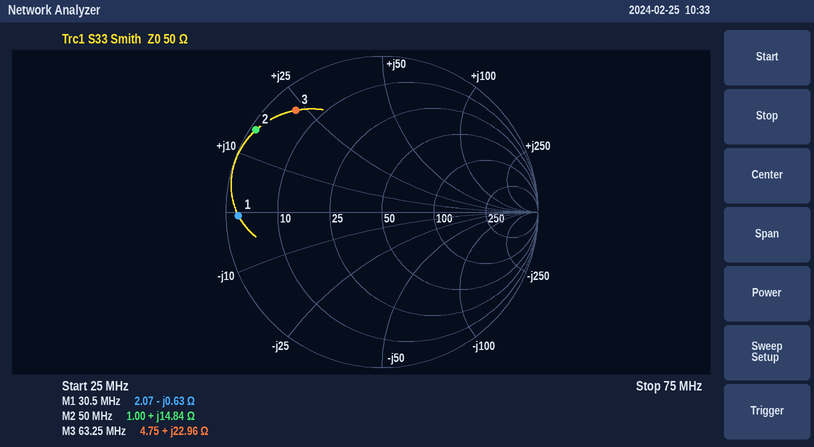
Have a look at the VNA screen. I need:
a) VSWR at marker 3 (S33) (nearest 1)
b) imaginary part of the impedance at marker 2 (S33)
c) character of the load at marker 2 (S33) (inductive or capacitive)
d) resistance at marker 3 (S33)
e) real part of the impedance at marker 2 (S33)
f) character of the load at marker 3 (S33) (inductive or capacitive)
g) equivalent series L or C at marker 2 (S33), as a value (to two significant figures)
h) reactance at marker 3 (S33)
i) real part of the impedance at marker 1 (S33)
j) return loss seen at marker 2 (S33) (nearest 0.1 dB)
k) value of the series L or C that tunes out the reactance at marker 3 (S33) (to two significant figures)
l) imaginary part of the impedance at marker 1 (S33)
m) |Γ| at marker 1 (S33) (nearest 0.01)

13
+14.84 Ω
inductive
4.75 Ω
1.00 Ω
inductive
47 nH
+22.96 Ω
2.07 Ω
0.3 dB
110 pF
-0.63 Ω
0.92
